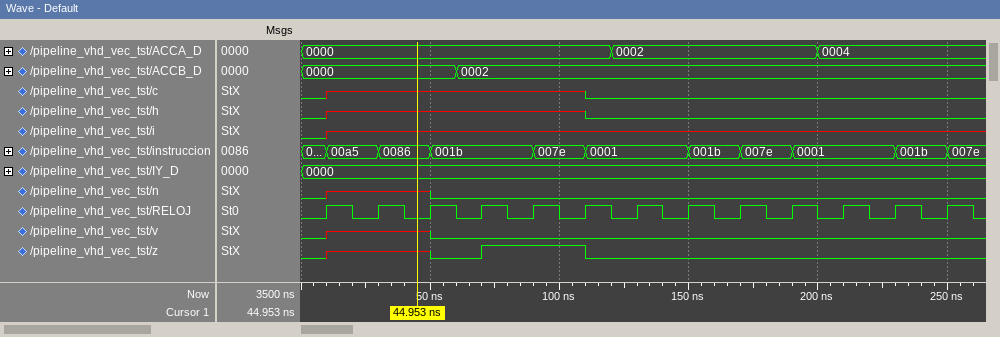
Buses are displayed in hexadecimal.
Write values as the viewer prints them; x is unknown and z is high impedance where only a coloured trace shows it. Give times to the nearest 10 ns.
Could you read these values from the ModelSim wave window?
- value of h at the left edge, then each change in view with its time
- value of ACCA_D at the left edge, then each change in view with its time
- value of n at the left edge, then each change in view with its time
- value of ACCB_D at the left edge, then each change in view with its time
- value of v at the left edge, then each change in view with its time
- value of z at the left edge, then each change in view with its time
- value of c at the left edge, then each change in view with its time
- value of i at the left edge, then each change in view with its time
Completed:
0, x at 10 ns, 0 at 110 ns
0000, 0002 at 120 ns, 0004 at 200 ns
0, x at 10 ns, 0 at 50 ns
0000, 0002 at 60 ns
0, x at 10 ns, 0 at 50 ns
0, x at 10 ns, 0 at 50 ns, 1 at 70 ns, 0 at 110 ns
0, x at 10 ns, 0 at 110 ns
0, x at 10 ns
